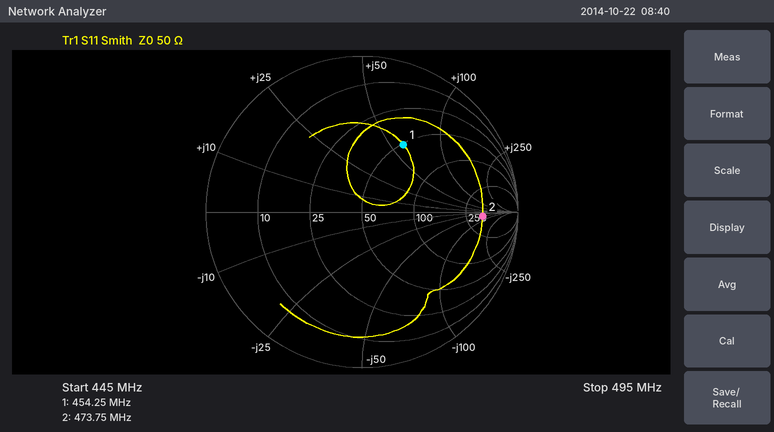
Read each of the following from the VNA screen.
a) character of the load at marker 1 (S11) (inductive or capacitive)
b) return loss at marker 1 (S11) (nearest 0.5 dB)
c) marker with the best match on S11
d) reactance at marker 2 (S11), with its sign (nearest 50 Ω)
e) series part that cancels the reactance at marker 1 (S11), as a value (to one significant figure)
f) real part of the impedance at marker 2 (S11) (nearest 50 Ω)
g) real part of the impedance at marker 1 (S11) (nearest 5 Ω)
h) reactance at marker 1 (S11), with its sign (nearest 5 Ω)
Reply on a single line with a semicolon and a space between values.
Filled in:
inductive; 6.0 dB; marker 1; -50 Ω; 6 pF; 400 Ω; 50 Ω; +60 Ω
